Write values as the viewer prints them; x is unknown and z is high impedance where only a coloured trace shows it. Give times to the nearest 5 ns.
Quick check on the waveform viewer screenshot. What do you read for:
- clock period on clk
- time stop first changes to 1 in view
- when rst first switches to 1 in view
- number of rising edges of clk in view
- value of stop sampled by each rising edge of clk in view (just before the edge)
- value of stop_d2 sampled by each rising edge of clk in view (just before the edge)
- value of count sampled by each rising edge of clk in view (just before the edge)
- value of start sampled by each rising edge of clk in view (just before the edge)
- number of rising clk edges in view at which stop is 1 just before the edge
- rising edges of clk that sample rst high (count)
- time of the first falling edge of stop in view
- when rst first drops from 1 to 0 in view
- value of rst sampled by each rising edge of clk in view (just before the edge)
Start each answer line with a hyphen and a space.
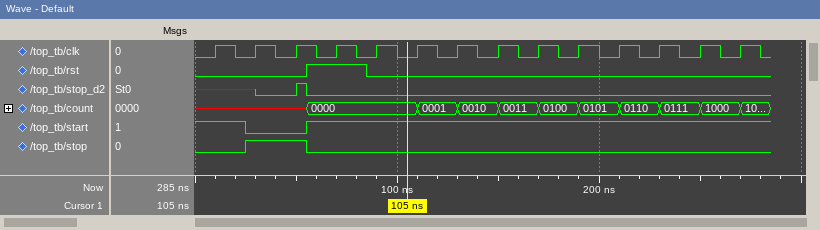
- 20 ns
- 25 ns
- 55 ns
- 14
- 0 1 1 0 0 0 0 0 0 0 0 0 0 0
- x x 0 0 0 0 0 0 0 0 0 0 0 0
- x, x, x, 0000, 0000, 0000, 0001, 0010, 0011, 0100, 0101, 0110, 0111, 1000
- 1 0 0 1 1 1 1 1 1 1 1 1 1 1
- 2
- 1
- 55 ns
- 85 ns
- 0 0 0 1 0 0 0 0 0 0 0 0 0 0
